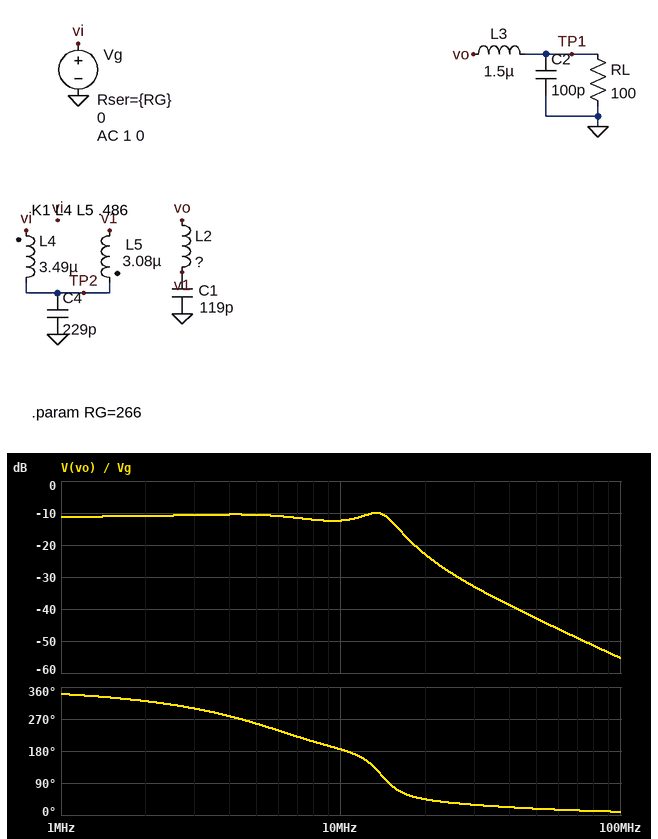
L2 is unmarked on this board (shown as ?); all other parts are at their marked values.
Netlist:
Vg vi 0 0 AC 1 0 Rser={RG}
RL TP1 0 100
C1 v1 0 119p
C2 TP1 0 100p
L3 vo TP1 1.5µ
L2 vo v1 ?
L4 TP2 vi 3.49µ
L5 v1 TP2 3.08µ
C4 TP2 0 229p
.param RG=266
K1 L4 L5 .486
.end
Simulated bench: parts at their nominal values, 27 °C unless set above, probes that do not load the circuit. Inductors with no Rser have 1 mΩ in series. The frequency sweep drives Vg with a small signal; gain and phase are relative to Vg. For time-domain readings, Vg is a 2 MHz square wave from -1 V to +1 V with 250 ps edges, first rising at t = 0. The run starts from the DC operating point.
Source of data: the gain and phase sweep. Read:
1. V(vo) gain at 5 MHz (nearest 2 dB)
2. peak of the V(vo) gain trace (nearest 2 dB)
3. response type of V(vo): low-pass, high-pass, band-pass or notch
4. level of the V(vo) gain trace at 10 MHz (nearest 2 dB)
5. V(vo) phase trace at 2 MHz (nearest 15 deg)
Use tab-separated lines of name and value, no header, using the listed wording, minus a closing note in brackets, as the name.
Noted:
V(vo) gain at 5 MHz	-10 dB
peak of the V(vo) gain trace	-10 dB
response type of V(vo): low-pass, high-pass, band-pass or notch	low-pass
level of the V(vo) gain trace at 10 MHz	-12 dB
V(vo) phase trace at 2 MHz	315 deg
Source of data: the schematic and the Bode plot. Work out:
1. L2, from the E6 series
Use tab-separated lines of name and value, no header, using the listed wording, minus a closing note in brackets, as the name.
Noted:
L2, from the E6 series	2.2 µH
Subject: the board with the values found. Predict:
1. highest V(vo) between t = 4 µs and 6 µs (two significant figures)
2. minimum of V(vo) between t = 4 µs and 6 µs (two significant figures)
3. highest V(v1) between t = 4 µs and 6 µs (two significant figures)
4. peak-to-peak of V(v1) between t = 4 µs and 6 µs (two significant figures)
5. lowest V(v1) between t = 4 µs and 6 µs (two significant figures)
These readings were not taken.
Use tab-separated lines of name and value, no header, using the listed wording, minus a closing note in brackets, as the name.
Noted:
highest V(vo) between t = 4 µs and 6 µs	370 mV
minimum of V(vo) between t = 4 µs and 6 µs	-370 mV
highest V(v1) between t = 4 µs and 6 µs	610 mV
peak-to-peak of V(v1) between t = 4 µs and 6 µs	1.2 V
lowest V(v1) between t = 4 µs and 6 µs	-610 mV
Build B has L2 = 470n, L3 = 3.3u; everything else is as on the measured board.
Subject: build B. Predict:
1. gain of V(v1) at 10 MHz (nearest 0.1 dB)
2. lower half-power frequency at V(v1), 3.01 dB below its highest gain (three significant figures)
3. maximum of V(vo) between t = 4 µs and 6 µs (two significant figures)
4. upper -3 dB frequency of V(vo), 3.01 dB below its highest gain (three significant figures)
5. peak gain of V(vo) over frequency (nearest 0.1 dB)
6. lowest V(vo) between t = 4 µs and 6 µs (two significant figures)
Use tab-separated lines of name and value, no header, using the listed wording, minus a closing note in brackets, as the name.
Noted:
gain of V(v1) at 10 MHz	-5.0 dB
lower half-power frequency at V(v1), 3.01 dB below its highest gain	10.8 MHz
maximum of V(vo) between t = 4 µs and 6 µs	530 mV
upper -3 dB frequency of V(vo), 3.01 dB below its highest gain	15.4 MHz
peak gain of V(vo) over frequency	-2.4 dB
lowest V(vo) between t = 4 µs and 6 µs	-530 mV
